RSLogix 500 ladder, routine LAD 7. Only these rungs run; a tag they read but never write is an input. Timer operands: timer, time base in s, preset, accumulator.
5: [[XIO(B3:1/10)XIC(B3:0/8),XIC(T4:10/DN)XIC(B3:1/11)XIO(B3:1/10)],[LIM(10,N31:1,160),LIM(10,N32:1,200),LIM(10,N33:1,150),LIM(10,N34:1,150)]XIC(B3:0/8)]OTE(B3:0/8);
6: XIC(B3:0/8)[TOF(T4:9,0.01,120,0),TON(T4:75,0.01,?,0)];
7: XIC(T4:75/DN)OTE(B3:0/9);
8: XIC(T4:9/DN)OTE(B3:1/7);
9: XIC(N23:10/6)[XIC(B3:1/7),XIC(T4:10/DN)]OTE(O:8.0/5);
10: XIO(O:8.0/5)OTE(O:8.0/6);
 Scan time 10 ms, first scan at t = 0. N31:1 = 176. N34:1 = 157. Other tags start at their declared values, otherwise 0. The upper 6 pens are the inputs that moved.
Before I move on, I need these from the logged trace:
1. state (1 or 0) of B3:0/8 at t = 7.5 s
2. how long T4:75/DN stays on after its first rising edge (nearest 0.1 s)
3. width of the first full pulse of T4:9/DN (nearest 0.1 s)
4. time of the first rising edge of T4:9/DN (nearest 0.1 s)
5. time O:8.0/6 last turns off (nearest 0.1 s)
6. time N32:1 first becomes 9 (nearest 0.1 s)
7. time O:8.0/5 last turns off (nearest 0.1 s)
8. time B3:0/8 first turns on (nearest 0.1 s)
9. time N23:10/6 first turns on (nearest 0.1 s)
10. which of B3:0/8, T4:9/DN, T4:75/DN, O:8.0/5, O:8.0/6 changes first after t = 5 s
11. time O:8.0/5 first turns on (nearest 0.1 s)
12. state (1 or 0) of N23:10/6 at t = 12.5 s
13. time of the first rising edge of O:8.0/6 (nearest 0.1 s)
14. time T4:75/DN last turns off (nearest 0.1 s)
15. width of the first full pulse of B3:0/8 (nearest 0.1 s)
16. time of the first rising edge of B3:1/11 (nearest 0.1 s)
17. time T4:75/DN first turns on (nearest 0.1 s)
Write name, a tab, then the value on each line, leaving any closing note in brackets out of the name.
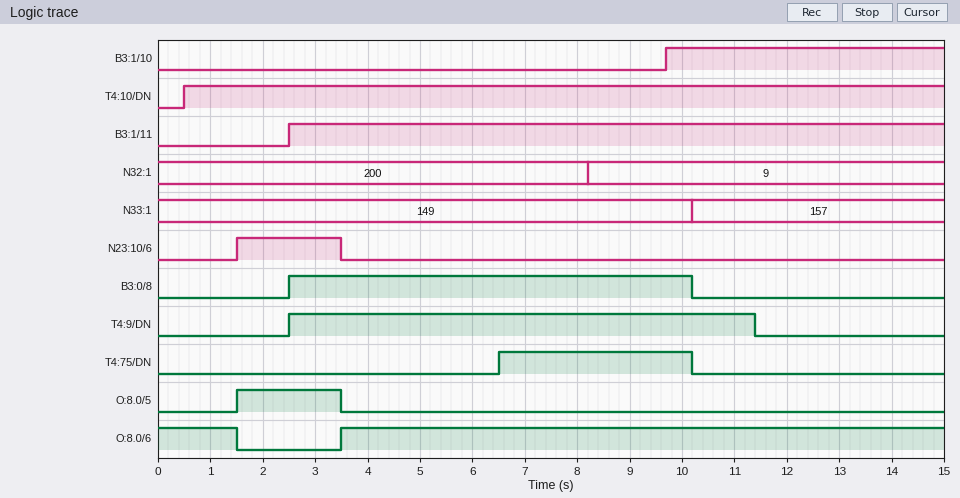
state (1 or 0) of B3:0/8 at t = 7.5 s	1
how long T4:75/DN stays on after its first rising edge	3.7 s
width of the first full pulse of T4:9/DN	8.9 s
time of the first rising edge of T4:9/DN	2.5 s
time O:8.0/6 last turns off	1.5 s
time N32:1 first becomes 9	8.2 s
time O:8.0/5 last turns off	3.5 s
time B3:0/8 first turns on	2.5 s
time N23:10/6 first turns on	1.5 s
which of B3:0/8, T4:9/DN, T4:75/DN, O:8.0/5, O:8.0/6 changes first after t = 5 s	T4:75/DN
time O:8.0/5 first turns on	1.5 s
state (1 or 0) of N23:10/6 at t = 12.5 s	0
time of the first rising edge of O:8.0/6	3.5 s
time T4:75/DN last turns off	10.2 s
width of the first full pulse of B3:0/8	7.7 s
time of the first rising edge of B3:1/11	2.5 s
time T4:75/DN first turns on	6.5 s
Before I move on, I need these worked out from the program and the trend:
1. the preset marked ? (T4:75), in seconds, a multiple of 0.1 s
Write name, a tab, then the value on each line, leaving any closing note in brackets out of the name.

the preset marked ? (T4:75), in seconds, a multiple of 0.1 s	4.0 s
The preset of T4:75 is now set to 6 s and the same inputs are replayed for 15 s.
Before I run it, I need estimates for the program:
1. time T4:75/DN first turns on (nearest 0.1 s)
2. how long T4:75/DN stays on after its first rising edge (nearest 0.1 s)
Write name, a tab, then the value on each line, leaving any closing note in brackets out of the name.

time T4:75/DN first turns on	8.5 s
how long T4:75/DN stays on after its first rising edge	1.7 s
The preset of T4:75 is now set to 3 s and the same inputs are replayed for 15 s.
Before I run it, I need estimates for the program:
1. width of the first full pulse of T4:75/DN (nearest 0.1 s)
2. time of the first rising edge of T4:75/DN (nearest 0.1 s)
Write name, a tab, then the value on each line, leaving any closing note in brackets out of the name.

width of the first full pulse of T4:75/DN	4.7 s
time of the first rising edge of T4:75/DN	5.5 s
